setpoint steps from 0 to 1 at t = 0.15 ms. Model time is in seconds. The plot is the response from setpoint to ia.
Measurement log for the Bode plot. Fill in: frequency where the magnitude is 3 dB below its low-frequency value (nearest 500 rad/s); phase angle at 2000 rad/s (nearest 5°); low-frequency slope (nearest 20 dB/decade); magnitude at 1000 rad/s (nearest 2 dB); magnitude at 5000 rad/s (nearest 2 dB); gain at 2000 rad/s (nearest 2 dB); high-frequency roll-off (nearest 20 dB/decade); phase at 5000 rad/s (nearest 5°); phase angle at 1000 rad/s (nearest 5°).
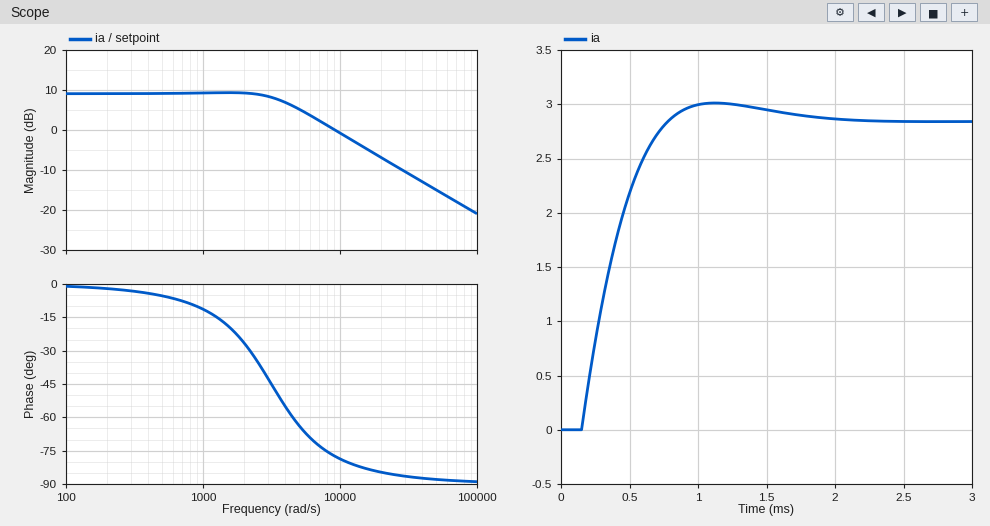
4500 rad/s
-25°
0 dB/decade
10 dB
6 dB
10 dB
-20 dB/decade
-65°
-10°
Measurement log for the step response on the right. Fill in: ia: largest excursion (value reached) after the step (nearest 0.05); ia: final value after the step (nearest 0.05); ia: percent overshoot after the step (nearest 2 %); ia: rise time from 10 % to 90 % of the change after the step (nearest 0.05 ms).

3.00
2.85
6 %
0.45 ms
